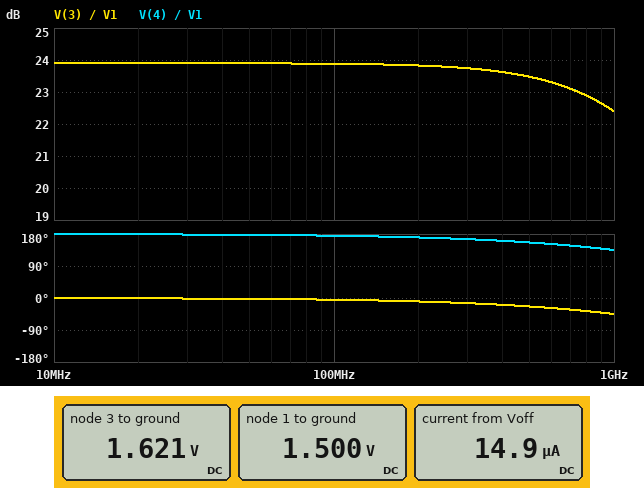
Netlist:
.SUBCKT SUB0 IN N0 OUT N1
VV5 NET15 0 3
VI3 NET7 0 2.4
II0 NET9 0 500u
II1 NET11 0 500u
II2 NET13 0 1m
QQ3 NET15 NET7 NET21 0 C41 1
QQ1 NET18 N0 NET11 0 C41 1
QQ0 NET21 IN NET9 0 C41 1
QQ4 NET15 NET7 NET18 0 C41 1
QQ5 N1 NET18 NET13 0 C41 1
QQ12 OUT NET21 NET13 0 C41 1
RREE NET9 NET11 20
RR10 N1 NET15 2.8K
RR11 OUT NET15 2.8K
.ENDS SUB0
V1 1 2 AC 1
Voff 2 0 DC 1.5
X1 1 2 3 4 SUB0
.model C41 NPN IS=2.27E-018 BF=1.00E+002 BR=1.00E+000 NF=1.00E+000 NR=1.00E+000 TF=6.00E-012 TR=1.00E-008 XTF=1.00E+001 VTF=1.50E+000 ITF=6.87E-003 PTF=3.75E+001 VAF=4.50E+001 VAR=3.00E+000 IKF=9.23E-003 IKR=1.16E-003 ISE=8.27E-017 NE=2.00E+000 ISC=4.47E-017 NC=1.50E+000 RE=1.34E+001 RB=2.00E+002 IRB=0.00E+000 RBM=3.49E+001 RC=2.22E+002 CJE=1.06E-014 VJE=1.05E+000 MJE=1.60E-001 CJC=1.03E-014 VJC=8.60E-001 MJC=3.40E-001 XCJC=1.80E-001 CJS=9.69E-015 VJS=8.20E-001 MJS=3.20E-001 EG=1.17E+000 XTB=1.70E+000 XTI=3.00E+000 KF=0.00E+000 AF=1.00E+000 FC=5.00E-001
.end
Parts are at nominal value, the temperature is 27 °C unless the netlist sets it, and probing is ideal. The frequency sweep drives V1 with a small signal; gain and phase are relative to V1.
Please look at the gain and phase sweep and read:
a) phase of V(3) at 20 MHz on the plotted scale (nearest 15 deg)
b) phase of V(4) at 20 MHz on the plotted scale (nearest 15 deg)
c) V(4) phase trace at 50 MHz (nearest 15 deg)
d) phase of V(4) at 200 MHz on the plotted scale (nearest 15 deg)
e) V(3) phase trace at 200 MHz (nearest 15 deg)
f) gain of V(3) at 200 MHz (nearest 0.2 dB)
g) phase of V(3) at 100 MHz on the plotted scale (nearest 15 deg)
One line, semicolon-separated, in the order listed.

0 deg; 180 deg; 180 deg; 165 deg; -15 deg; 23.8 dB; 0 deg
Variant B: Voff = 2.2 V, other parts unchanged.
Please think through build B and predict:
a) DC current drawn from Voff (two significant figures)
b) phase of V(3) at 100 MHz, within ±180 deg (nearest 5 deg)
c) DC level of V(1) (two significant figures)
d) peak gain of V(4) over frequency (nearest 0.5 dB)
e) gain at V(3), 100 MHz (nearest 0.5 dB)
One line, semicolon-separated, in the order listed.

56 µA; -95 deg; 2.2 V; 18.0 dB; 10.0 dB
